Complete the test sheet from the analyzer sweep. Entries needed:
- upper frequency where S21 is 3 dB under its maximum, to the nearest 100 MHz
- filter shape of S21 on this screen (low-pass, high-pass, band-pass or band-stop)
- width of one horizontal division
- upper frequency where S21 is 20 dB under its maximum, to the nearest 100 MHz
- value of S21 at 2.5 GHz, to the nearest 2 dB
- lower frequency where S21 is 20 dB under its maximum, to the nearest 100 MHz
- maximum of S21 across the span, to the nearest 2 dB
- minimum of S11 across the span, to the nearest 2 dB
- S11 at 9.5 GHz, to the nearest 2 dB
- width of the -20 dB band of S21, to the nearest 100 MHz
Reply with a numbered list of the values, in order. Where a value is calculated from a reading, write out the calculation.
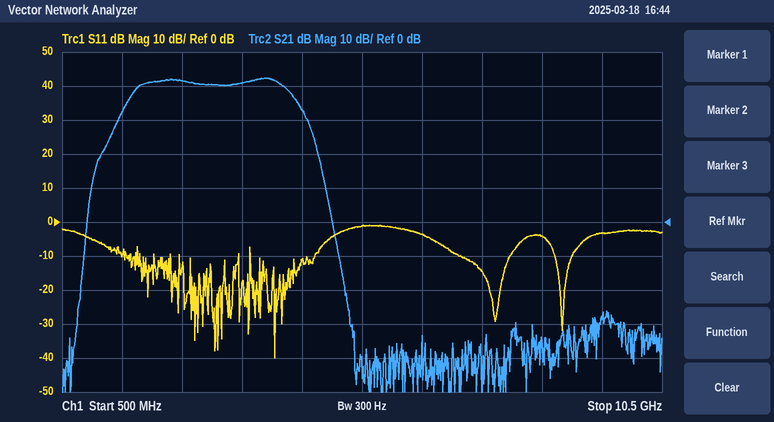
1. 4.2 GHz
2. band-pass
3. 1 GHz
4. 4.7 GHz
5. 42 dB
6. 1.2 GHz
7. 42 dB
8. -40 dB
9. -4 dB
10. 4.7 GHz − 1.2 GHz = 3.5 GHz
